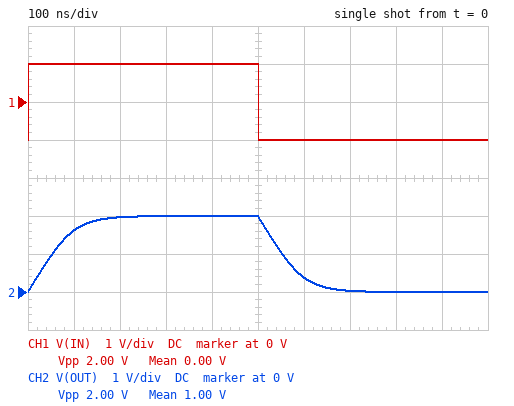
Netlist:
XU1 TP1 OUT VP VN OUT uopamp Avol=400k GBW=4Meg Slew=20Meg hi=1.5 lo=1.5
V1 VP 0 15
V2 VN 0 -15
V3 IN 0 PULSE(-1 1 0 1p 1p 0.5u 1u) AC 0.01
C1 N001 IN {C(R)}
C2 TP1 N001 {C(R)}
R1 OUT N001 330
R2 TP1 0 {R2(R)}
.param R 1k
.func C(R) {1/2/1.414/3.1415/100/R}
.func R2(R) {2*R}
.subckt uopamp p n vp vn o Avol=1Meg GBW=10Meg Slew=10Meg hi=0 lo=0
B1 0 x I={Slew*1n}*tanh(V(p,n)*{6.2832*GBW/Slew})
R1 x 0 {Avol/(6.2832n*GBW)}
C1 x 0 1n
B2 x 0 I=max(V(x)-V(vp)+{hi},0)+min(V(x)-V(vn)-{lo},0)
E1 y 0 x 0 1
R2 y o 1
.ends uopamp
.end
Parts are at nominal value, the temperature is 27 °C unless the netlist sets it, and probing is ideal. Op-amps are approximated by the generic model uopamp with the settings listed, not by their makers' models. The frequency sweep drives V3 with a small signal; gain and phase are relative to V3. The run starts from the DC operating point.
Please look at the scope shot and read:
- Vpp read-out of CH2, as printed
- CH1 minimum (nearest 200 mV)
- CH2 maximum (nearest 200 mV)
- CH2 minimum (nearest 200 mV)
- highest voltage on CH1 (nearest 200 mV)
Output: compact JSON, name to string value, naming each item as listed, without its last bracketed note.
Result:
{"Vpp read-out of CH2, as printed": "2.00 V", "CH1 minimum": "-1.0 V", "CH2 maximum": "2.0 V", "CH2 minimum": "0 V", "highest voltage on CH1": "1.0 V"}
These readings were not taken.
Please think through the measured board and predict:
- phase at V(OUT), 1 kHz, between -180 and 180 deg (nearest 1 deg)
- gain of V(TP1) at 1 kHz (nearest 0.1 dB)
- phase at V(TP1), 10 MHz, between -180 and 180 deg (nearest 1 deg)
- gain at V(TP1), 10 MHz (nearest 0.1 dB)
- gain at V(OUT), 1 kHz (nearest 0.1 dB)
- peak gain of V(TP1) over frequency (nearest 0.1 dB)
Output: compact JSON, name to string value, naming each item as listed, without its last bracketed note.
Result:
{"phase at V(OUT), 1 kHz, between -180 and 180 deg": "8 deg", "gain of V(TP1) at 1 kHz": "0.2 dB", "phase at V(TP1), 10 MHz, between -180 and 180 deg": "0 deg", "gain at V(TP1), 10 MHz": "0 dB", "gain at V(OUT), 1 kHz": "0.2 dB", "peak gain of V(TP1) over frequency": "2.6 dB"}
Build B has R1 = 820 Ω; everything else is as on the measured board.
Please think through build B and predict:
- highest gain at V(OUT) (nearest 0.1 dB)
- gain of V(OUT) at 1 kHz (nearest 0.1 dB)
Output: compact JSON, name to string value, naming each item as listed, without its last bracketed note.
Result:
{"highest gain at V(OUT)": "0.1 dB", "gain of V(OUT) at 1 kHz": "0 dB"}
